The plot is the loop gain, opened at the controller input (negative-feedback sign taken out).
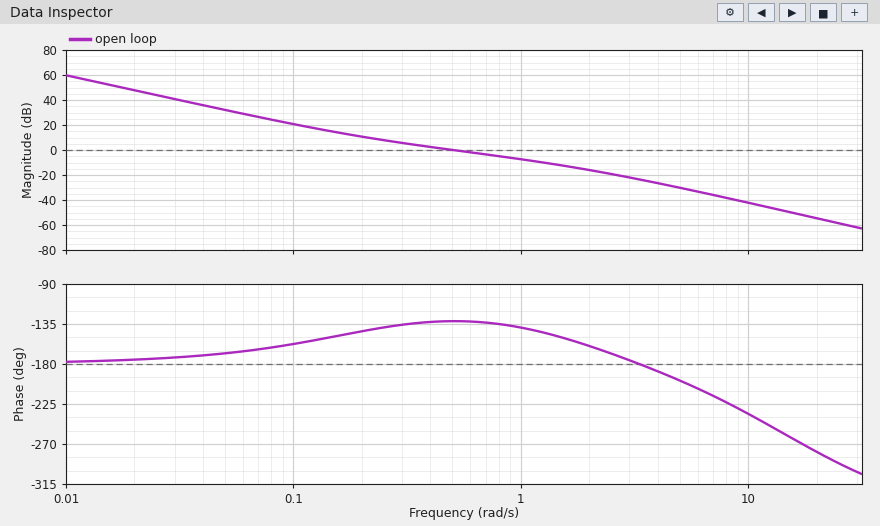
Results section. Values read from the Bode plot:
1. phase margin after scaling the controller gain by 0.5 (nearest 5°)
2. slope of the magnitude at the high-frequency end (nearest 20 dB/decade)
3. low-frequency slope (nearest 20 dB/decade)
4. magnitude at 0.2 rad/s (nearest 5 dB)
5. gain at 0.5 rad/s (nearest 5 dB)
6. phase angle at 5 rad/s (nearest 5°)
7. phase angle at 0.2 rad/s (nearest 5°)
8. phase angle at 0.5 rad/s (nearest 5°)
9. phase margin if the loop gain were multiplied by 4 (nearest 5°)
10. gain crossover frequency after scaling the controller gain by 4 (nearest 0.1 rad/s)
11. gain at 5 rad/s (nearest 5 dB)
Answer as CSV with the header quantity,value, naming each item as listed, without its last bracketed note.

quantity,value
phase margin after scaling the controller gain by 0.5,45°
slope of the magnitude at the high-frequency end,-40 dB/decade
low-frequency slope,-40 dB/decade
magnitude at 0.2 rad/s,10 dB
gain at 0.5 rad/s,0 dB
phase angle at 5 rad/s,-200°
phase angle at 0.2 rad/s,-145°
phase angle at 0.5 rad/s,-130°
phase margin if the loop gain were multiplied by 4,30°
gain crossover frequency after scaling the controller gain by 4,1.5 rad/s
gain at 5 rad/s,-30 dB
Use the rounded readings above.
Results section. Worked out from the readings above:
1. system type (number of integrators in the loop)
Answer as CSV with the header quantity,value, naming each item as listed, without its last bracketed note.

quantity,value
system type,2
